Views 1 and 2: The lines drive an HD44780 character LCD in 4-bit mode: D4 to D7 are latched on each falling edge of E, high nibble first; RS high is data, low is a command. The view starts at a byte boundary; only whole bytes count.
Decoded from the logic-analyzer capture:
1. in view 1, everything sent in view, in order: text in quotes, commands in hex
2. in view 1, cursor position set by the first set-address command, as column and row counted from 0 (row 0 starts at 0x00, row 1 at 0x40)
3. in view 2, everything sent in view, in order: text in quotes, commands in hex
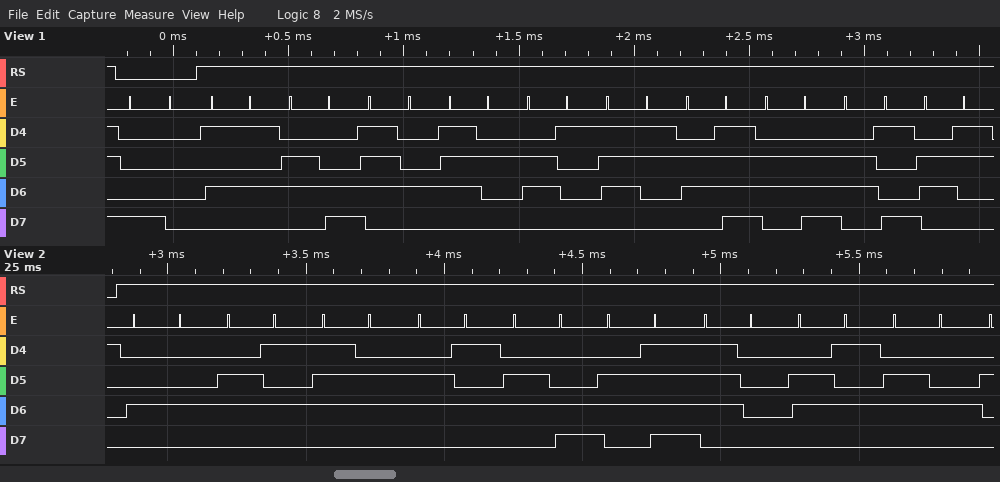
0x80 "Ultrasonic"
column 0, row 0
"Developed"
